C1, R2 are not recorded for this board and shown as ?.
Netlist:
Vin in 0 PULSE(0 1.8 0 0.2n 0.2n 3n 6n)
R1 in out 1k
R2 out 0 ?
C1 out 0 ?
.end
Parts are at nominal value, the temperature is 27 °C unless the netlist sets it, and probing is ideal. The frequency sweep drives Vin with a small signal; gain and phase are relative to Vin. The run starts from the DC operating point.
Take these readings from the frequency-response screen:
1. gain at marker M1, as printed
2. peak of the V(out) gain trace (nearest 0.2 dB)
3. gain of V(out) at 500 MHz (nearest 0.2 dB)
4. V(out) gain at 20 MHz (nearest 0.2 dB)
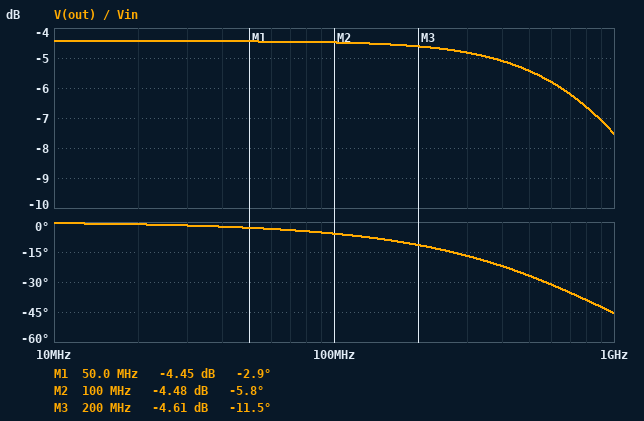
-4.45 dB
-4.4 dB
-5.4 dB
-4.4 dB
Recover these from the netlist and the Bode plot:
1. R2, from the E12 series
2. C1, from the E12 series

1.5 kΩ
270 fF
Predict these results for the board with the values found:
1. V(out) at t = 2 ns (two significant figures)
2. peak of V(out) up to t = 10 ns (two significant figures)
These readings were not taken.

1.1 V
1.1 V
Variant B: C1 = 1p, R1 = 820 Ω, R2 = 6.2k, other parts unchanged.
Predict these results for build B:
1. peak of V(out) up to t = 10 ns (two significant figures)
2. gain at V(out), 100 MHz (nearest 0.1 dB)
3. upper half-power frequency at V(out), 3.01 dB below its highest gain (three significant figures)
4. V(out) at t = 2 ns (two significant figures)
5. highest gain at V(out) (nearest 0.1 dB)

1.6 V
-1.9 dB
220 MHz
1.5 V
-1.1 dB
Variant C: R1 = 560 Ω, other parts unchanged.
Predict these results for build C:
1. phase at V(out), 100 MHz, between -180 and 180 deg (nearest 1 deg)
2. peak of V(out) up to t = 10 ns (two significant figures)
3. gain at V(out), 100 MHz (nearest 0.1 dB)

-4 deg
1.3 V
-2.8 dB
